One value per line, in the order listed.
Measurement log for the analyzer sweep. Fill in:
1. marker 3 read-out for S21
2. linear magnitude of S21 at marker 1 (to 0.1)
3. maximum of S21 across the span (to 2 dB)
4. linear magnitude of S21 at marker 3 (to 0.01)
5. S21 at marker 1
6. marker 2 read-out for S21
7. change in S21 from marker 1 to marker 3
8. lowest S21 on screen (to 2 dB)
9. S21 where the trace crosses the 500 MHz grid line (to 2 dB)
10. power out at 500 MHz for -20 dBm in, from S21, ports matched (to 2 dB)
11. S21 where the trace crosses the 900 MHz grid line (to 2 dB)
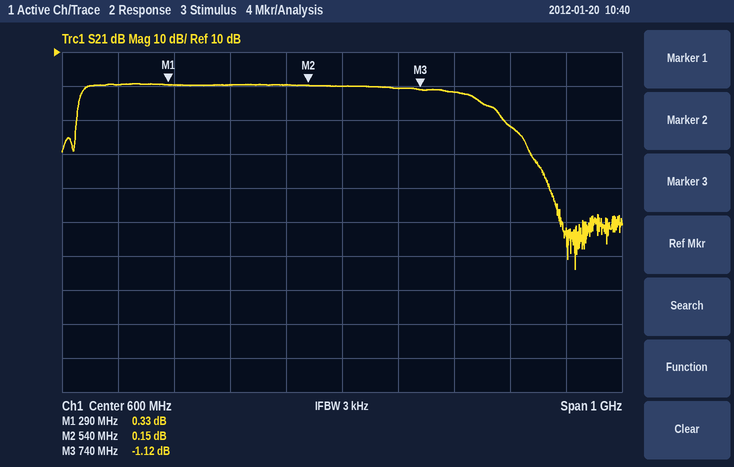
-1.12 dB
1.0
0 dB
0.88
0.33 dB
0.15 dB
-1.45 dB
-54 dB
0 dB
-20 dBm
-12 dB
